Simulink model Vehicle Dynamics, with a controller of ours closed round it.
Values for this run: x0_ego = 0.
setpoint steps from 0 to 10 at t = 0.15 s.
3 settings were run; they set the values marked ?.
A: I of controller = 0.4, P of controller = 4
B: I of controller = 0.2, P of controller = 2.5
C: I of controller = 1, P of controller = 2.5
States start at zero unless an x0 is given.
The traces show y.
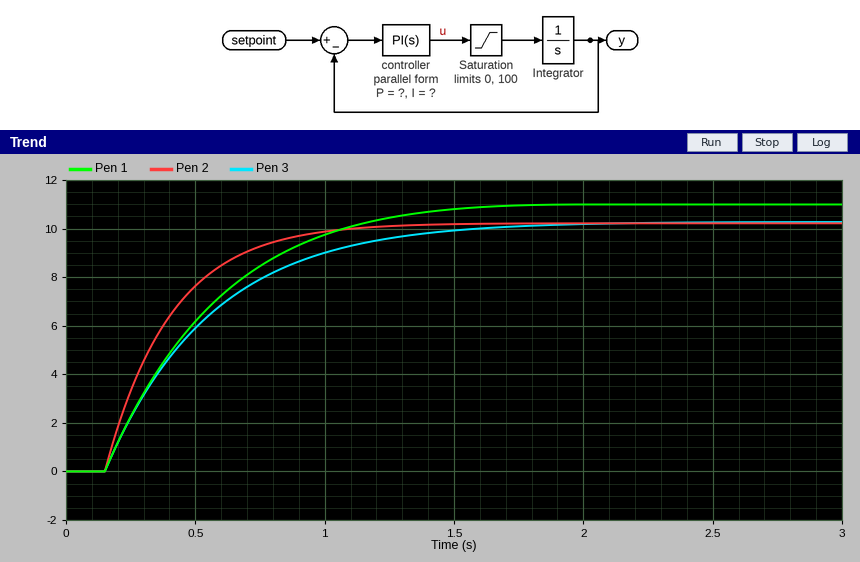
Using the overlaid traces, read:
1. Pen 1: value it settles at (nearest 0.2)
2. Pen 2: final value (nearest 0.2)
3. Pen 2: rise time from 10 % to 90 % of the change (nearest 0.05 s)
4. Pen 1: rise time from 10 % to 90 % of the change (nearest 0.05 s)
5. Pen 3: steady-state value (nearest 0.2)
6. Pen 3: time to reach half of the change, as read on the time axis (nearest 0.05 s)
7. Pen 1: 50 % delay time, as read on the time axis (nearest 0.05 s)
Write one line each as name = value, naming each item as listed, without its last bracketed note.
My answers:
Pen 1: value it settles at = 11.0
Pen 2: final value = 10.2
Pen 2: rise time from 10 % to 90 % of the change = 0.55 s
Pen 1: rise time from 10 % to 90 % of the change = 0.85 s
Pen 3: steady-state value = 10.2
Pen 3: time to reach half of the change, as read on the time axis = 0.45 s
Pen 1: 50 % delay time, as read on the time axis = 0.45 s
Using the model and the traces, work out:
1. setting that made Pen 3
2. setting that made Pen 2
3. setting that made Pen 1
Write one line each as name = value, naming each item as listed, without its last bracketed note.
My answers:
setting that made Pen 3 = B
setting that made Pen 2 = A
setting that made Pen 1 = C
